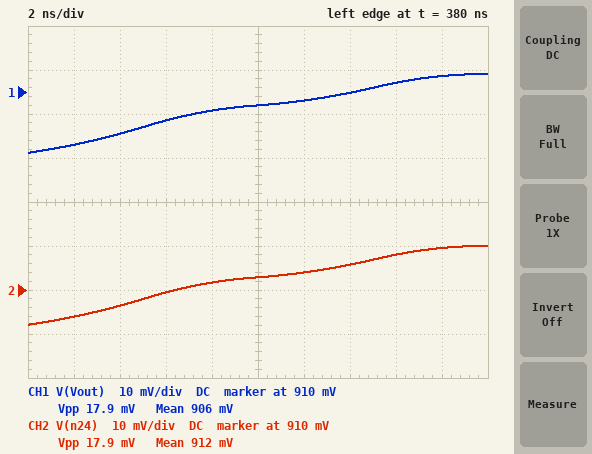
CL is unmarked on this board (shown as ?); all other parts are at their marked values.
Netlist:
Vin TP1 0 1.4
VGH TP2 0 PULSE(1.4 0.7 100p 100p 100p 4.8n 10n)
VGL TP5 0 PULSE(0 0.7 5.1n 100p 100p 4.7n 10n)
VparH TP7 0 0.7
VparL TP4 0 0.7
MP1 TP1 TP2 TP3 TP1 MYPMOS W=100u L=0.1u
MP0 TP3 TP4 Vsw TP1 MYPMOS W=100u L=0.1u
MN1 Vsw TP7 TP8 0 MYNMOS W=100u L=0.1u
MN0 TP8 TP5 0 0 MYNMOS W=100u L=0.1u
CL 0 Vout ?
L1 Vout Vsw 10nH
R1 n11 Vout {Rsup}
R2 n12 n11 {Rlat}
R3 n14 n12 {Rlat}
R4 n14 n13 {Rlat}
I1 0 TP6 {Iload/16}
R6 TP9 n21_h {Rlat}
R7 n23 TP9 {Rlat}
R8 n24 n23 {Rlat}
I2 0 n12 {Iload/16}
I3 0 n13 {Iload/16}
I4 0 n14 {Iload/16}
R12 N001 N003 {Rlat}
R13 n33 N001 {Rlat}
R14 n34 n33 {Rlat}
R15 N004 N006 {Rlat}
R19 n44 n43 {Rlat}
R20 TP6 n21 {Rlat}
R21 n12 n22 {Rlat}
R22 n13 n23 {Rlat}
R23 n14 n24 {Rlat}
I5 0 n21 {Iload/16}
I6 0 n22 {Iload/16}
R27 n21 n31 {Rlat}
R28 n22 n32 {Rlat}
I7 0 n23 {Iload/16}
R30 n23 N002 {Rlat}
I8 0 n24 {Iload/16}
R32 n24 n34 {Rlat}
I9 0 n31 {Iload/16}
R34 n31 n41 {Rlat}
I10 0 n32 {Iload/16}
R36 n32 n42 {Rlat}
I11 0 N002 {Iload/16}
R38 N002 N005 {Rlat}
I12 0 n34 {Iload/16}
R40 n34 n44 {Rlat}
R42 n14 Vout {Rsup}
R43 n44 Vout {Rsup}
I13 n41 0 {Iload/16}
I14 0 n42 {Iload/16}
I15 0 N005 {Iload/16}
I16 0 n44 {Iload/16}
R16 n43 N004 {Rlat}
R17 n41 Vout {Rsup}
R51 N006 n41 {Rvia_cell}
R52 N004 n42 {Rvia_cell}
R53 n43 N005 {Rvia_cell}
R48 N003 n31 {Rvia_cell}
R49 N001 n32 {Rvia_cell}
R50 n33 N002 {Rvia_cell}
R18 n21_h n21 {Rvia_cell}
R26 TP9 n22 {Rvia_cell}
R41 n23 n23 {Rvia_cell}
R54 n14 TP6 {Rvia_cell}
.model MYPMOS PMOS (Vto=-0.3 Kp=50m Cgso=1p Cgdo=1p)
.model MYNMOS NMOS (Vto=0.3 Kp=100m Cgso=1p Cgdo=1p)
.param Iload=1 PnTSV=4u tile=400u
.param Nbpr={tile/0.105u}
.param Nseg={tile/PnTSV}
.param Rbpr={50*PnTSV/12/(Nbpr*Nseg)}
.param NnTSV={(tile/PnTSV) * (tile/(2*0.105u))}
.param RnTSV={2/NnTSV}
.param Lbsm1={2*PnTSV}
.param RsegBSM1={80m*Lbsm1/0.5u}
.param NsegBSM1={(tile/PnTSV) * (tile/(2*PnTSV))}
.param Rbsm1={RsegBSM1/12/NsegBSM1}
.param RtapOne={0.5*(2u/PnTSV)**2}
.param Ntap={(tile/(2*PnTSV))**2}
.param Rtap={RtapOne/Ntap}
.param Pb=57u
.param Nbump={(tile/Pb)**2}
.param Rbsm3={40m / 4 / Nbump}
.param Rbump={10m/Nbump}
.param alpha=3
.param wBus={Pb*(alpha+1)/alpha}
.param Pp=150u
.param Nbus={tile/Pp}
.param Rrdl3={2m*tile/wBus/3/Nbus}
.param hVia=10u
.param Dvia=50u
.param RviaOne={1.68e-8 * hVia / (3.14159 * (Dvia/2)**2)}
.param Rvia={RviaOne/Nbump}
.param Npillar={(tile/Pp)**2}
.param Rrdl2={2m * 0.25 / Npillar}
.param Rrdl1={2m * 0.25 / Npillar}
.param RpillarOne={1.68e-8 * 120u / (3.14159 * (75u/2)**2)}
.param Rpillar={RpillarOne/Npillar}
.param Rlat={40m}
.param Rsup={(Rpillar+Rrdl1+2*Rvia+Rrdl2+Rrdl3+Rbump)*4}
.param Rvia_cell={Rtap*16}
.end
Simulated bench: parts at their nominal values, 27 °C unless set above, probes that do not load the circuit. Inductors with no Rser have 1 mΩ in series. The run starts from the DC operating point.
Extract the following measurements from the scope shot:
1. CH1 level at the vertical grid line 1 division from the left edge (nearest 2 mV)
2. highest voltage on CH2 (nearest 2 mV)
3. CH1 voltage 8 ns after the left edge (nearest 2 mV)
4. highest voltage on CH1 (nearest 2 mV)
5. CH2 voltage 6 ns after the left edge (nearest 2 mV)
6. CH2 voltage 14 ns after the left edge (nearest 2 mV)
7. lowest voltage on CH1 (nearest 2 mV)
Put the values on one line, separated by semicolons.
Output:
898 mV; 920 mV; 906 mV; 914 mV; 910 mV; 916 mV; 896 mV
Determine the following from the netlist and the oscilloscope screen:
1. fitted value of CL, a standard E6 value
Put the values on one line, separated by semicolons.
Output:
330 nF
